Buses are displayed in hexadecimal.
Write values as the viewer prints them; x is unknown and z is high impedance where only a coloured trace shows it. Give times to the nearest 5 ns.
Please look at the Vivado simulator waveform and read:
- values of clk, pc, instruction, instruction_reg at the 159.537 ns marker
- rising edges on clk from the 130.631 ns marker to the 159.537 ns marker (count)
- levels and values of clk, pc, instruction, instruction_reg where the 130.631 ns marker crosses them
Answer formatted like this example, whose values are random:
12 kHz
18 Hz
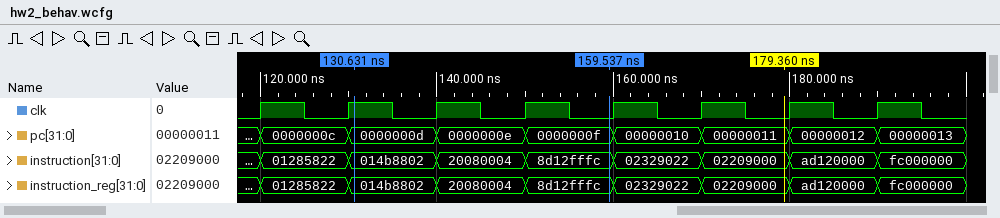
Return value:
clk=0, pc=0000000f, instruction=8d12fffc, instruction_reg=8d12fffc
2
clk=1, pc=0000000d, instruction=014b8802, instruction_reg=014b8802
